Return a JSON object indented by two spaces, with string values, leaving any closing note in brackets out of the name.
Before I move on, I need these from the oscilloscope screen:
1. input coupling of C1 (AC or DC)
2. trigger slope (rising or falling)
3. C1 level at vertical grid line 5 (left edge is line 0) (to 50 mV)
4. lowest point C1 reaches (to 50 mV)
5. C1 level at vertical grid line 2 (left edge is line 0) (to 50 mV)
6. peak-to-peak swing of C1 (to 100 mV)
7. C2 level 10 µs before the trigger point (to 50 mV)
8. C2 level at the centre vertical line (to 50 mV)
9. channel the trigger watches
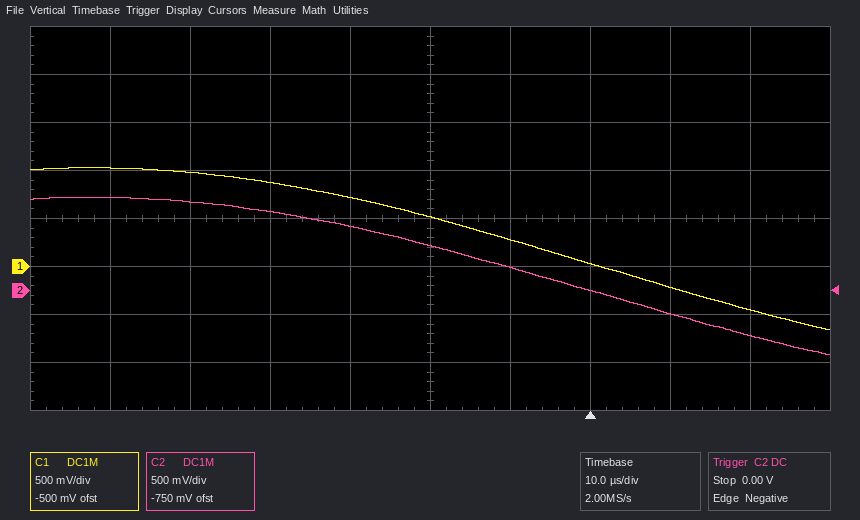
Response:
{
  "input coupling of C1": "DC",
  "trigger slope": "falling",
  "C1 level at vertical grid line 5 (left edge is line 0)": "500 mV",
  "lowest point C1 reaches": "-650 mV",
  "C1 level at vertical grid line 2 (left edge is line 0)": "1.00 V",
  "peak-to-peak swing of C1": "1.70 V",
  "C2 level 10 µs before the trigger point": "250 mV",
  "C2 level at the centre vertical line": "450 mV",
  "channel the trigger watches": "C2"
}
